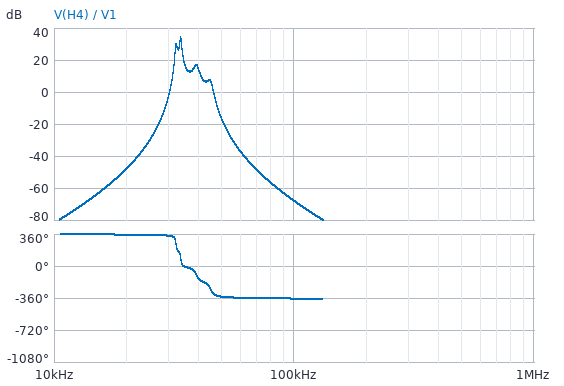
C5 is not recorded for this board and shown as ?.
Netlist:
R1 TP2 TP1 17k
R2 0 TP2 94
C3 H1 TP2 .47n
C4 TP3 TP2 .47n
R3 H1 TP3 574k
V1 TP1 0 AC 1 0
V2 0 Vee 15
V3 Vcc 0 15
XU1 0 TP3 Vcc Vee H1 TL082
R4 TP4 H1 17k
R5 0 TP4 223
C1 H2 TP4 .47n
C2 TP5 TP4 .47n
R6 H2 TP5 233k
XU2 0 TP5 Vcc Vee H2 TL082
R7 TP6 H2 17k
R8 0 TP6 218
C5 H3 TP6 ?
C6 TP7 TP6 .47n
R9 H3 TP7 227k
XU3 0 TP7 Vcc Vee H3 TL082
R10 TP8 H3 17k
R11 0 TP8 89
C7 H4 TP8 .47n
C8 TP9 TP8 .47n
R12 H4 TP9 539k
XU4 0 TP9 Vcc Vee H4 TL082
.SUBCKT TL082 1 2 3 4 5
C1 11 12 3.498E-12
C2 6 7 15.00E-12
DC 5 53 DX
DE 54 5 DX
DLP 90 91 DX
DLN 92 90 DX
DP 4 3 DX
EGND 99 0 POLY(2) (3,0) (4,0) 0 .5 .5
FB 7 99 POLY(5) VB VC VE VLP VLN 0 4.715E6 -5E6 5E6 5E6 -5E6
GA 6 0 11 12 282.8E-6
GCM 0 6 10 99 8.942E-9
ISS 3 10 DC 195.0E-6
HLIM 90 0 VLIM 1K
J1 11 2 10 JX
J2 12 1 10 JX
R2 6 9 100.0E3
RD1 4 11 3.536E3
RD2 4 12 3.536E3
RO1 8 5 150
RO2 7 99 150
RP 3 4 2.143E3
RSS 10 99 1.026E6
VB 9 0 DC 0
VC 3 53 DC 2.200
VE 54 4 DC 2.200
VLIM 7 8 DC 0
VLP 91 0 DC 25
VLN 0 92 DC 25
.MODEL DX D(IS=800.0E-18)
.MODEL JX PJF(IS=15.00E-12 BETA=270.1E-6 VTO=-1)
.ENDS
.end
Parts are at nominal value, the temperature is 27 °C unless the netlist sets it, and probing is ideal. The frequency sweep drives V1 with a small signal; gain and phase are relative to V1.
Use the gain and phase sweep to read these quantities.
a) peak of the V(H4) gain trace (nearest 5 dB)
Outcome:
35 dB
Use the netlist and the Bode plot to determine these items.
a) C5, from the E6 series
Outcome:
330 pF
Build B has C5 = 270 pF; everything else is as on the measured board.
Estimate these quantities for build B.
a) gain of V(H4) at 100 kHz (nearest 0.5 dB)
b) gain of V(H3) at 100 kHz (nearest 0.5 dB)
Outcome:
-66.5 dB
-47.0 dB
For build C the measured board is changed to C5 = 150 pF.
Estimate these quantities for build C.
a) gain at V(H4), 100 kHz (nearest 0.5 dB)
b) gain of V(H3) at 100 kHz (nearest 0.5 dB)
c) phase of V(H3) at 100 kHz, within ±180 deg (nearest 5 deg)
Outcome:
-63.5 dB
-44.0 dB
-95 deg
